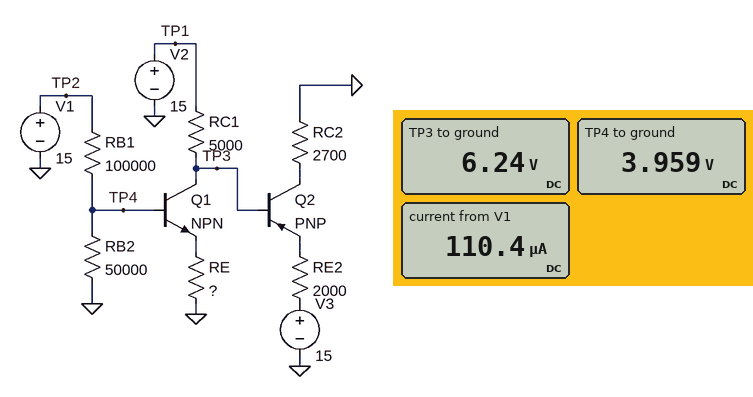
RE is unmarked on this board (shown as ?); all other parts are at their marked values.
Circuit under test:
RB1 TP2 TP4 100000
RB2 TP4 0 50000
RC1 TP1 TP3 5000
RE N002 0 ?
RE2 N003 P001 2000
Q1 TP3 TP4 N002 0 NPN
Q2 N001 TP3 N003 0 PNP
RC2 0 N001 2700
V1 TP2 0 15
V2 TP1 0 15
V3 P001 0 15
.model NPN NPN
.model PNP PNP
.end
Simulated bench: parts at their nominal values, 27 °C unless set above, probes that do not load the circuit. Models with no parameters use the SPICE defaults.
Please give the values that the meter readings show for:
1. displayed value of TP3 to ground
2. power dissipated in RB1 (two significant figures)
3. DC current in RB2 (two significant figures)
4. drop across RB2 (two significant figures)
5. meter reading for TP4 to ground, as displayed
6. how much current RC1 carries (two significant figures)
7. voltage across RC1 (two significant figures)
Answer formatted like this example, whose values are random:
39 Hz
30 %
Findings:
6.24 V
1.2 mW
79 µA
4.0 V
3.959 V
1.8 mA
8.8 V
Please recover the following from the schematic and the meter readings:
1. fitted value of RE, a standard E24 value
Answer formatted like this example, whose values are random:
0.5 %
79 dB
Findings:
1 kΩ
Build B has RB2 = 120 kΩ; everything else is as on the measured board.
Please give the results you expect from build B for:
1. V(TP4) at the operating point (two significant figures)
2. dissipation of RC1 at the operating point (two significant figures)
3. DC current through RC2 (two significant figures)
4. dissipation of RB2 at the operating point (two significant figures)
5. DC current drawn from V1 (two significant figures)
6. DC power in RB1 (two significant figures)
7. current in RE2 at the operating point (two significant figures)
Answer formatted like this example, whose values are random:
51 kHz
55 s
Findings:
5.5 V
21 mW
2.1 mA
250 µW
95 µA
910 µW
4.7 mA
